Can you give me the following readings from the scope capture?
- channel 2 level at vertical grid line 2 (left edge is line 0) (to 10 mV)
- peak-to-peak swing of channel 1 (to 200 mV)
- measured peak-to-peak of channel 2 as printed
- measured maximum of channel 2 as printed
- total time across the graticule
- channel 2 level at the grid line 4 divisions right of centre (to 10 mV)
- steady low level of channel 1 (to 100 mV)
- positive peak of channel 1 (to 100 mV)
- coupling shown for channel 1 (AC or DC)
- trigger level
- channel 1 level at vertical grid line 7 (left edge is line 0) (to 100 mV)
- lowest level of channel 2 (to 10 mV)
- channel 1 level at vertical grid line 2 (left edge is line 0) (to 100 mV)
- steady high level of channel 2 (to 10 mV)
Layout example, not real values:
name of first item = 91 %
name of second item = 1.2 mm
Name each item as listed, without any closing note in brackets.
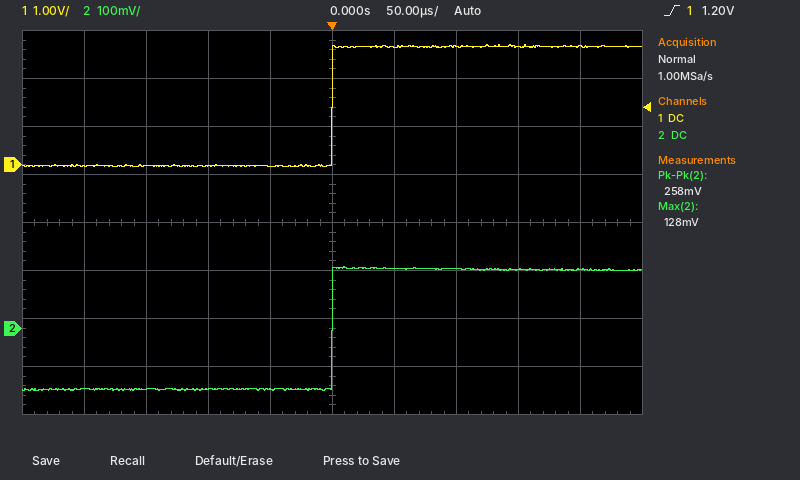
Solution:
channel 2 level at vertical grid line 2 (left edge is line 0) = -130 mV
peak-to-peak swing of channel 1 = 2.6 V
measured peak-to-peak of channel 2 as printed = 258 mV
measured maximum of channel 2 as printed = 128 mV
total time across the graticule = 500 µs
channel 2 level at the grid line 4 divisions right of centre = 120 mV
steady low level of channel 1 = 0.0 V
positive peak of channel 1 = 2.5 V
coupling shown for channel 1 = DC
trigger level = 1.20 V
channel 1 level at vertical grid line 7 (left edge is line 0) = 2.5 V
lowest level of channel 2 = -130 mV
channel 1 level at vertical grid line 2 (left edge is line 0) = 0.0 V
steady high level of channel 2 = 120 mV
